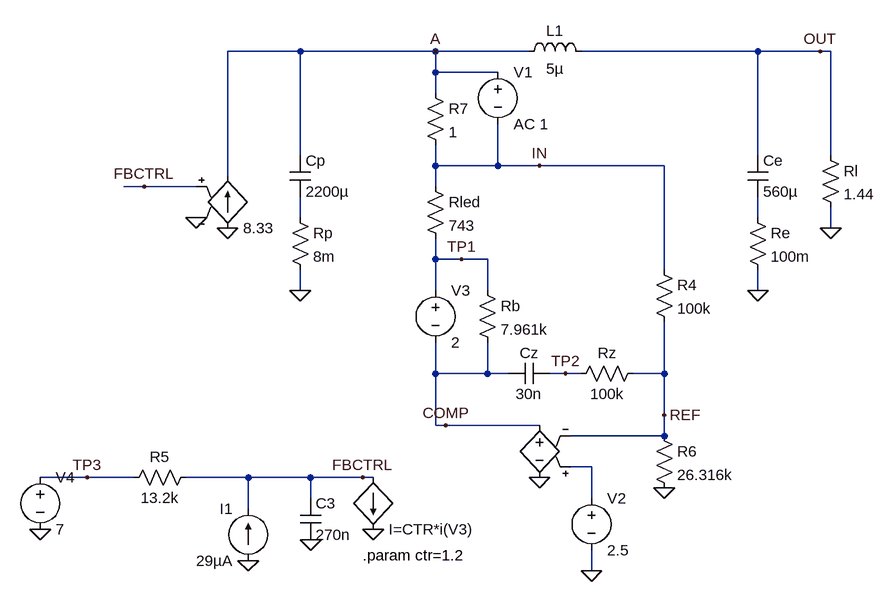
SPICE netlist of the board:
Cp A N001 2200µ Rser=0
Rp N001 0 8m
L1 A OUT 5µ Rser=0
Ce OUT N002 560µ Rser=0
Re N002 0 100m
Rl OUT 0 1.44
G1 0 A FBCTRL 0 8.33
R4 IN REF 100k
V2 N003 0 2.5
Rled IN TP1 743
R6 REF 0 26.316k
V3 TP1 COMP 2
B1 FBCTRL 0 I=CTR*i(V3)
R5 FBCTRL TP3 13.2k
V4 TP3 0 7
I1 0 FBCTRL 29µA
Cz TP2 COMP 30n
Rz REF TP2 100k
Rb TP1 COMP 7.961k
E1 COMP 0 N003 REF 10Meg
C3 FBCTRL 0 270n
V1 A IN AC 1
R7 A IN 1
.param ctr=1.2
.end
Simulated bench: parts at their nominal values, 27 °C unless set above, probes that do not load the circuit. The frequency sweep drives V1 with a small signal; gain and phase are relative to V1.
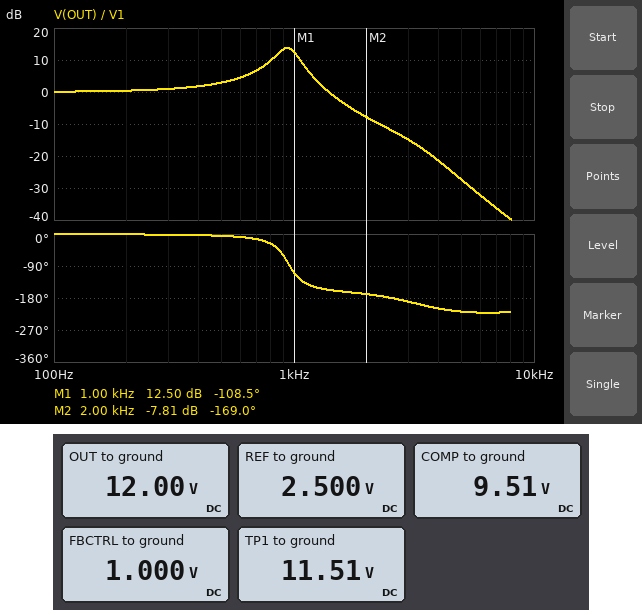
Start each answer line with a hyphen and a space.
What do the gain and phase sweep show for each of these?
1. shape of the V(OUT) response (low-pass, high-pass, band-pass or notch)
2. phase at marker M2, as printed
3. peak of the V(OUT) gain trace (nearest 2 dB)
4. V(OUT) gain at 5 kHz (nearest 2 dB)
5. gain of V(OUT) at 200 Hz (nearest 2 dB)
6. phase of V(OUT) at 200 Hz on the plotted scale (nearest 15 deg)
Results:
- low-pass
- -169.0 deg
- 14 dB
- -28 dB
- 0 dB
- 0 deg
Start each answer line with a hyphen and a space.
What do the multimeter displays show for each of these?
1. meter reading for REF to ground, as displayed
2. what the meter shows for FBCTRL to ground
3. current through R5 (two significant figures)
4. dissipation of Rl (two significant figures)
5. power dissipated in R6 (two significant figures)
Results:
- 2.500 V
- 1.000 V
- 450 µA
- 100 W
- 240 µW
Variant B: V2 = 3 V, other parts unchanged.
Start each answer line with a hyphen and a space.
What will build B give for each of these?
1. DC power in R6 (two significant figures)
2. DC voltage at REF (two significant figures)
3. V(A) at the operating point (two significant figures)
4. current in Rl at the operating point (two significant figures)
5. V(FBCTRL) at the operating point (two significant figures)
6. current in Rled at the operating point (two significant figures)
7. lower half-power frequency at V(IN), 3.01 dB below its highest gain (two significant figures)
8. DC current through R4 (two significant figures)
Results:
- 340 µW
- 3.0 V
- 14 V
- 10 A
- 1.2 V
- 640 µA
- 870 Hz
- 110 µA
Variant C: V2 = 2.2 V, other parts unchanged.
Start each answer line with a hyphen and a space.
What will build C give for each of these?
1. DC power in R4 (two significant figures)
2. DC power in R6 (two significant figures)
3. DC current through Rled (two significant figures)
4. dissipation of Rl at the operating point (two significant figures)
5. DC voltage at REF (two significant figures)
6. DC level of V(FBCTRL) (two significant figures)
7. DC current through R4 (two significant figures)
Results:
- 700 µW
- 180 µW
- 660 µA
- 77 W
- 2.2 V
- 880 mV
- 84 µA
